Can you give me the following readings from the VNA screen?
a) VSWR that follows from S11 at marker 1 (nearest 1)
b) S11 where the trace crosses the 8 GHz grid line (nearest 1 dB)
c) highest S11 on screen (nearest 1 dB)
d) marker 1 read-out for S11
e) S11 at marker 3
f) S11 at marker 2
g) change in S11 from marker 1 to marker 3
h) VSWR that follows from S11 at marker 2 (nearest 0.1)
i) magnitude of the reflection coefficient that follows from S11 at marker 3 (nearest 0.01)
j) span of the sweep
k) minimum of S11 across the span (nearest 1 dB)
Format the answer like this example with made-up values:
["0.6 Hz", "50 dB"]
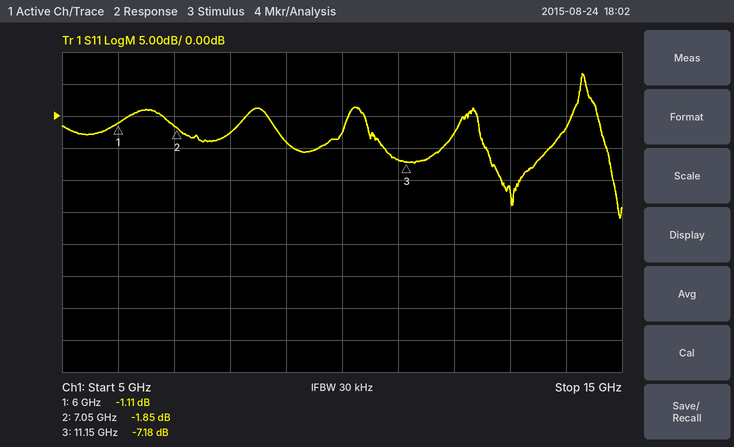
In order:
["16", "-3 dB", "7 dB", "-1.11 dB", "-7.18 dB", "-1.85 dB", "-6.07 dB", "9.4", "0.44", "10 GHz", "-16 dB"]
